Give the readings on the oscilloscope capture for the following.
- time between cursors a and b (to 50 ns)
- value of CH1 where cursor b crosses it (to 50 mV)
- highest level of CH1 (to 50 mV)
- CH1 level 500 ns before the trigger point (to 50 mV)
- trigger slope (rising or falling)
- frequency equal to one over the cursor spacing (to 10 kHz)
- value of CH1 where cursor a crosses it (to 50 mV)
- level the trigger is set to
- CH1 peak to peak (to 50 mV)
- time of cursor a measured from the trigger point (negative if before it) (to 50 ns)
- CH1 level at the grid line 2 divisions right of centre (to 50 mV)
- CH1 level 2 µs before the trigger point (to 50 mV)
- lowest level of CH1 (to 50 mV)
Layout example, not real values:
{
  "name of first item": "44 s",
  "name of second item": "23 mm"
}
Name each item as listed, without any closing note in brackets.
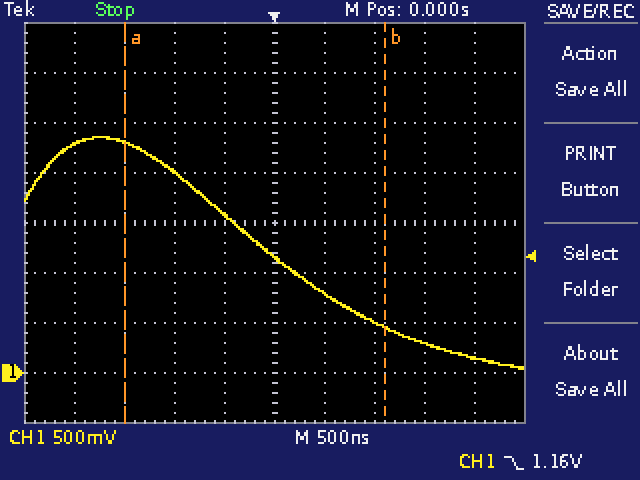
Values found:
{
  "time between cursors a and b": "2.60 µs",
  "value of CH1 where cursor b crosses it": "450 mV",
  "highest level of CH1": "2.35 V",
  "CH1 level 500 ns before the trigger point": "1.60 V",
  "trigger slope": "falling",
  "frequency equal to one over the cursor spacing": "380 kHz",
  "value of CH1 where cursor a crosses it": "2.30 V",
  "level the trigger is set to": "1.16 V",
  "CH1 peak to peak": "2.30 V",
  "time of cursor a measured from the trigger point (negative if before it)": "-1.50 µs",
  "CH1 level at the grid line 2 divisions right of centre": "500 mV",
  "CH1 level 2 µs before the trigger point": "2.30 V",
  "lowest level of CH1": "50 mV"
}
